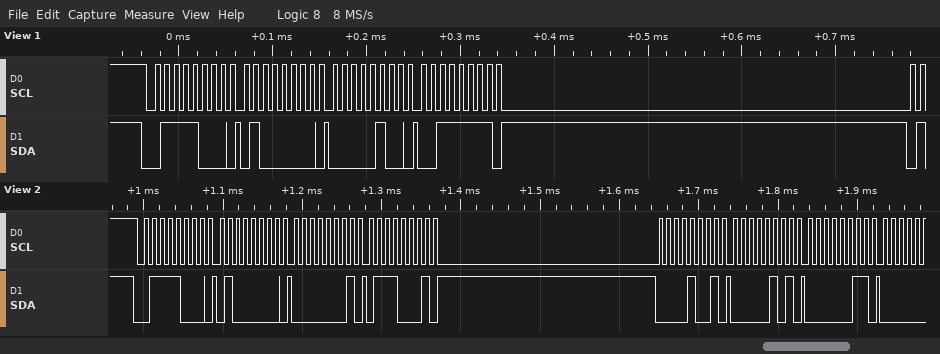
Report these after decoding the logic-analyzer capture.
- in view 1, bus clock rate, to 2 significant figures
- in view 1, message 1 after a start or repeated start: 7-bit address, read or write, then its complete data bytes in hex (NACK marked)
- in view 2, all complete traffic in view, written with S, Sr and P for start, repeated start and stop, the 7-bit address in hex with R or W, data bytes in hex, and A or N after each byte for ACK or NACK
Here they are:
100 kHz
0x3C write: 40 04 3F
S 3CW A 40 A 01 A 71 A 09 A 05 A 03 A
